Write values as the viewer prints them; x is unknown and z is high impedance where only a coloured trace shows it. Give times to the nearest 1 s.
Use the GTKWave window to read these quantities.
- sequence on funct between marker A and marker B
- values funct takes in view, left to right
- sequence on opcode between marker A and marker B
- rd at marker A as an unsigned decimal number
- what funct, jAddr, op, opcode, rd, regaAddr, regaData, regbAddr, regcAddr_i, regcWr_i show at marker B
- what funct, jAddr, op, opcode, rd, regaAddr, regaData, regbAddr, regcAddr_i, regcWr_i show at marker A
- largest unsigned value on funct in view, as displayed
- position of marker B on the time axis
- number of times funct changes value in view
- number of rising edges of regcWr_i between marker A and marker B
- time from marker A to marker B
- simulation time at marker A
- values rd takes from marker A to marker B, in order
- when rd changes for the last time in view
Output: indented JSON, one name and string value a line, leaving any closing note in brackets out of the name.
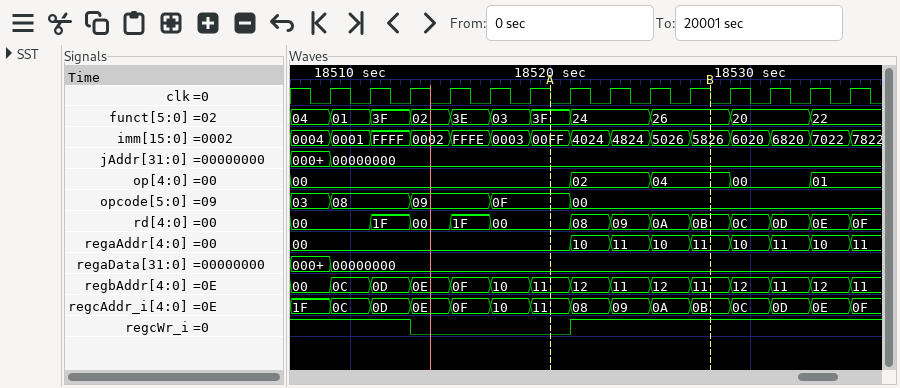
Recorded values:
{
  "sequence on funct between marker A and marker B": "3F, 24, 26",
  "values funct takes in view, left to right": "04, 01, 3F, 02, 3E, 03, 3F, 24, 26, 20, 22",
  "sequence on opcode between marker A and marker B": "0F, 00",
  "rd at marker A as an unsigned decimal number": "0",
  "what funct, jAddr, op, opcode, rd, regaAddr, regaData, regbAddr, regcAddr_i, regcWr_i show at marker B": "funct=26, jAddr=00000000, op=04, opcode=00, rd=0B, regaAddr=11, regaData=00000000, regbAddr=11, regcAddr_i=0B, regcWr_i=1",
  "what funct, jAddr, op, opcode, rd, regaAddr, regaData, regbAddr, regcAddr_i, regcWr_i show at marker A": "funct=3F, jAddr=00000000, op=00, opcode=0F, rd=00, regaAddr=00, regaData=00000000, regbAddr=11, regcAddr_i=11, regcWr_i=0",
  "largest unsigned value on funct in view, as displayed": "3F",
  "position of marker B on the time axis": "18528 s",
  "number of times funct changes value in view": "10",
  "number of rising edges of regcWr_i between marker A and marker B": "1",
  "time from marker A to marker B": "8 s",
  "simulation time at marker A": "18520 s",
  "values rd takes from marker A to marker B, in order": "00, 08, 09, 0A, 0B",
  "when rd changes for the last time in view": "18535 s"
}
